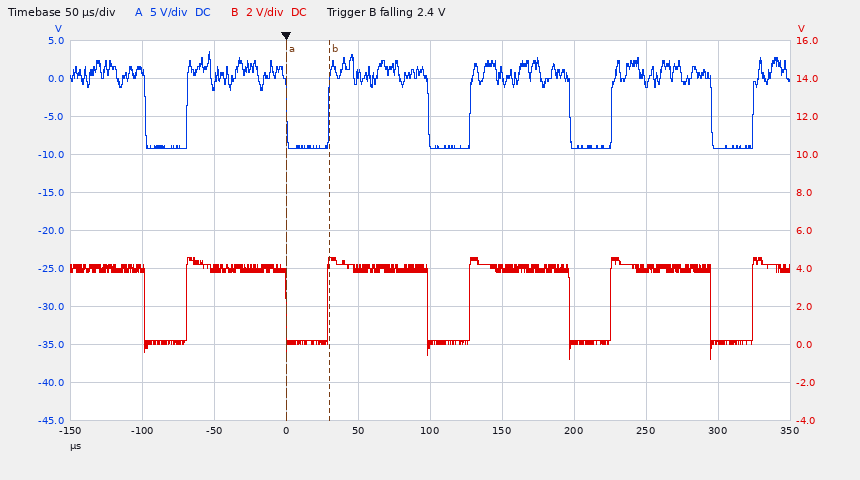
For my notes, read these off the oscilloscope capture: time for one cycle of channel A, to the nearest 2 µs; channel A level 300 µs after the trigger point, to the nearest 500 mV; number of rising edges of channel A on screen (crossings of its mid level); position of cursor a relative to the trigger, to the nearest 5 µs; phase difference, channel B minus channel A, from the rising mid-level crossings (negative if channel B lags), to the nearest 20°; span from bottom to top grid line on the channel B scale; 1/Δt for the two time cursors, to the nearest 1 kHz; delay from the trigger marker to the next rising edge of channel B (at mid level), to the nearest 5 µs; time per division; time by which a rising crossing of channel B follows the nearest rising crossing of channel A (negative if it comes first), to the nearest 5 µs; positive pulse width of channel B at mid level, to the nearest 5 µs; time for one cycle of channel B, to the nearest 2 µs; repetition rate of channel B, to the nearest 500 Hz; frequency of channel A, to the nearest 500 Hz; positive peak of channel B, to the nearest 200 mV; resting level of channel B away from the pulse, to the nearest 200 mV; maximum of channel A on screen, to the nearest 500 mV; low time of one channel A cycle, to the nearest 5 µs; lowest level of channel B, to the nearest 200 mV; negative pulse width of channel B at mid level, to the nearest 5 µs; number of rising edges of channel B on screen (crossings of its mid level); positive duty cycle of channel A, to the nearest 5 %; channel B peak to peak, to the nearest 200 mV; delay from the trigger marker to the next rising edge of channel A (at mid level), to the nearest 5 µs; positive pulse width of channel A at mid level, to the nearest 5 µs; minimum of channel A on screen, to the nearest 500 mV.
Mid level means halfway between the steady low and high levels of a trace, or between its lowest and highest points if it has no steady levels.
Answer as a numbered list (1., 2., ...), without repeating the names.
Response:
1. 98 µs
2. -9.0 V
3. 5
4. 0 µs
5. 0°
6. 20 V
7. 33 kHz
8. 30 µs
9. 50 µs
10. 0 µs
11. 70 µs
12. 98 µs
13. 10.0 kHz
14. 10.0 kHz
15. 4.6 V
16. 4.0 V
17. 3.5 V
18. 30 µs
19. -800 mV
20. 30 µs
21. 5
22. 70 %
23. 5.4 V
24. 30 µs
25. 70 µs
26. -9.0 V
